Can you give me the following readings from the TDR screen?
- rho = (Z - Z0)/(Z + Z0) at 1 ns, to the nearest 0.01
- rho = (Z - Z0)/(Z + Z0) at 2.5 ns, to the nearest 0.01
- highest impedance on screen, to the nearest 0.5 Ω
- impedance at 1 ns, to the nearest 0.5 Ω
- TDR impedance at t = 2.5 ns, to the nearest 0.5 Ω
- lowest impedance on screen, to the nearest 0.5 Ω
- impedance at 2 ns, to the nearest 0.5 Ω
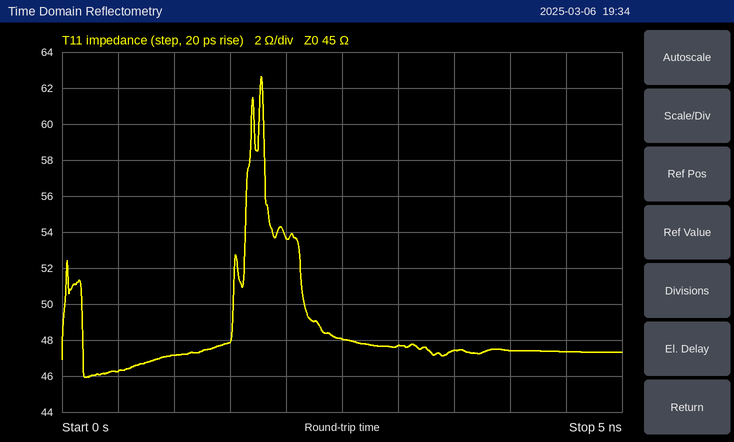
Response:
+0.02
+0.03
62.5 Ω
47.0 Ω
48.0 Ω
46.0 Ω
53.5 Ω
